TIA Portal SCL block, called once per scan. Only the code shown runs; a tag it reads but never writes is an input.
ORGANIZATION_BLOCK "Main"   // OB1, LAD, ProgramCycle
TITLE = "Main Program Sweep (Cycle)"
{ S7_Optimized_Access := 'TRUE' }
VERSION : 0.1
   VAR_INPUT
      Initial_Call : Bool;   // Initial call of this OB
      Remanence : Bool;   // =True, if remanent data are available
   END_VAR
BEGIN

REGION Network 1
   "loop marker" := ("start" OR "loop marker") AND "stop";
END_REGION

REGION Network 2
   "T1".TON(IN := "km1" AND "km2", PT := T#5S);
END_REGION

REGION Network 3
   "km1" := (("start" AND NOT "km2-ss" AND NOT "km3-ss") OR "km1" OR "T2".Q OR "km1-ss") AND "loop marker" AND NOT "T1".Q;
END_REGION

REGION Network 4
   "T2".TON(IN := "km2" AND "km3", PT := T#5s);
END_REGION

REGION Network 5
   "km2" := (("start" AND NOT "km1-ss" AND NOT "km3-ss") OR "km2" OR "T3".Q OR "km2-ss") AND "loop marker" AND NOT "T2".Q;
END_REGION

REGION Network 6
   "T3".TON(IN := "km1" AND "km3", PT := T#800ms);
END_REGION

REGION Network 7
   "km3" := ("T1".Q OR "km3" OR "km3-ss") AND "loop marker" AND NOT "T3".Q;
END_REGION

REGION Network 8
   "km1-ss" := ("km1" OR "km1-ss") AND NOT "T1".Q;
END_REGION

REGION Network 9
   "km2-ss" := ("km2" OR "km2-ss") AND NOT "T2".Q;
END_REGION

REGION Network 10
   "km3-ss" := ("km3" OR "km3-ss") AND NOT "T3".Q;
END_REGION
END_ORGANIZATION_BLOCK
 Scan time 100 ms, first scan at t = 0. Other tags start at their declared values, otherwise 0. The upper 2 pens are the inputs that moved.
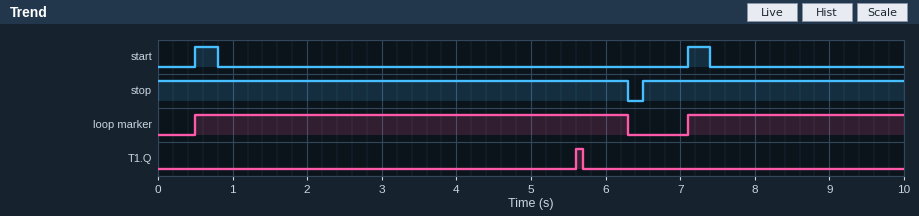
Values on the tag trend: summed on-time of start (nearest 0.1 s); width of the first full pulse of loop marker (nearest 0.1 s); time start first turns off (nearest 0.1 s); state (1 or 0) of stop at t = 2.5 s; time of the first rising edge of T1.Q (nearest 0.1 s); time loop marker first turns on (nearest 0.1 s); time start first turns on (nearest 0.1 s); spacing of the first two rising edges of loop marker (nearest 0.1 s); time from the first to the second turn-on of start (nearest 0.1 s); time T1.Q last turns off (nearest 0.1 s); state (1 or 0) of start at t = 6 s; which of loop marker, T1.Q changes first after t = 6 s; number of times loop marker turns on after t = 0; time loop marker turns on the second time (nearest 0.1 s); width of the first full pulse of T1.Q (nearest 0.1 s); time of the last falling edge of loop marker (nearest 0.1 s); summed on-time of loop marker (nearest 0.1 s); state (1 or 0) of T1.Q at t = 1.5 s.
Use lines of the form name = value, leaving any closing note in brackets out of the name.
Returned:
summed on-time of start = 0.6 s
width of the first full pulse of loop marker = 5.8 s
time start first turns off = 0.8 s
state (1 or 0) of stop at t = 2.5 s = 1
time of the first rising edge of T1.Q = 5.6 s
time loop marker first turns on = 0.5 s
time start first turns on = 0.5 s
spacing of the first two rising edges of loop marker = 6.6 s
time from the first to the second turn-on of start = 6.6 s
time T1.Q last turns off = 5.7 s
state (1 or 0) of start at t = 6 s = 0
which of loop marker, T1.Q changes first after t = 6 s = loop marker
number of times loop marker turns on after t = 0 = 2
time loop marker turns on the second time = 7.1 s
width of the first full pulse of T1.Q = 0.1 s
time of the last falling edge of loop marker = 6.3 s
summed on-time of loop marker = 8.7 s
state (1 or 0) of T1.Q at t = 1.5 s = 0
